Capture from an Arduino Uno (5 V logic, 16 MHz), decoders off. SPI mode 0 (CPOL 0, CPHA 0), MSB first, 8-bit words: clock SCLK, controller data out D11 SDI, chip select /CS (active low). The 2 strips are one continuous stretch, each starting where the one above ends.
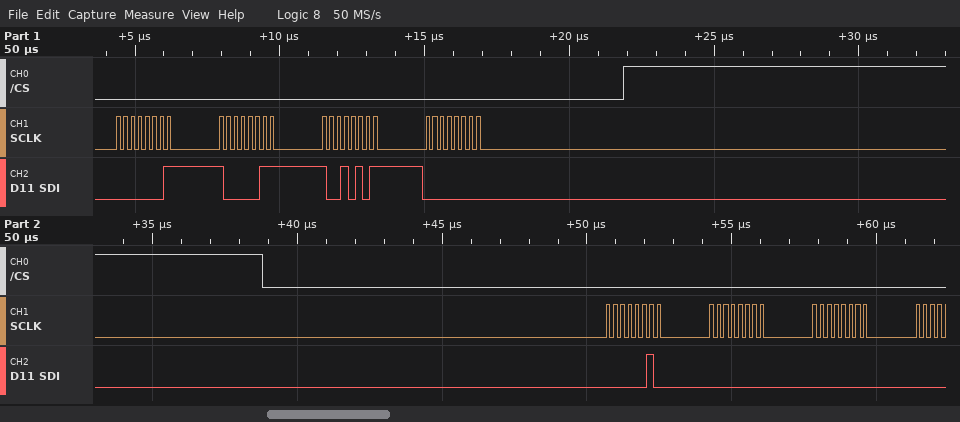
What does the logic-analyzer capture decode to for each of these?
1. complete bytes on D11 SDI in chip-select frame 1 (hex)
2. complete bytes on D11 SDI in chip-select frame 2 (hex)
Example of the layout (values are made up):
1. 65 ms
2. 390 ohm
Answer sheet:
1. 01 83 95 00
2. 02 00 00
